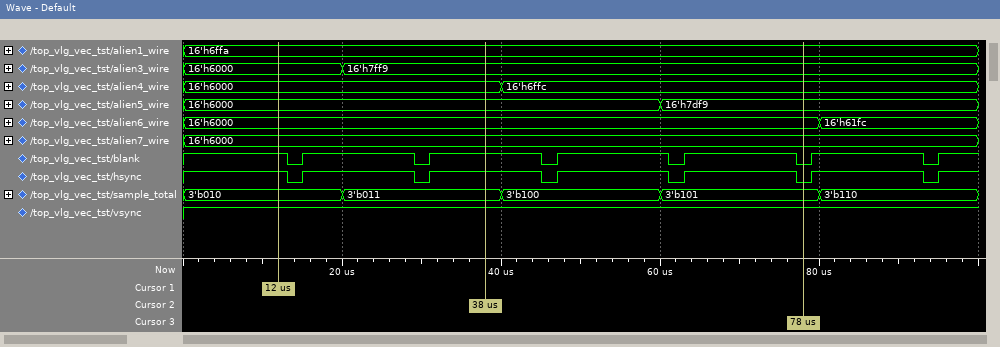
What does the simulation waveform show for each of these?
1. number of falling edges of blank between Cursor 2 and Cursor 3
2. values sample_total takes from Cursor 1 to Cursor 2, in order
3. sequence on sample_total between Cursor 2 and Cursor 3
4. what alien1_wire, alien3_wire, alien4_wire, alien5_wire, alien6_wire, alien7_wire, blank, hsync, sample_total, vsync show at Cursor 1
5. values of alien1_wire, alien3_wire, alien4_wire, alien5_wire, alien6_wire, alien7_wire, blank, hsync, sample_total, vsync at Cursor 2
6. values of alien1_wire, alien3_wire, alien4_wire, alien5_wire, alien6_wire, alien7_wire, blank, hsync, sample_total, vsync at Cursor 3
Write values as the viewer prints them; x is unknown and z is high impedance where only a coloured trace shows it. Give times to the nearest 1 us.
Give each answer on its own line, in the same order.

3
3'b010, 3'b011
3'b011, 3'b100, 3'b101
alien1_wire=16'h6ffa, alien3_wire=16'h6000, alien4_wire=16'h6000, alien5_wire=16'h6000, alien6_wire=16'h6000, alien7_wire=16'h6000, blank=1, hsync=1, sample_total=3'b010, vsync=1
alien1_wire=16'h6ffa, alien3_wire=16'h7ff9, alien4_wire=16'h6000, alien5_wire=16'h6000, alien6_wire=16'h6000, alien7_wire=16'h6000, blank=1, hsync=1, sample_total=3'b011, vsync=1
alien1_wire=16'h6ffa, alien3_wire=16'h7ff9, alien4_wire=16'h6ffc, alien5_wire=16'h7df9, alien6_wire=16'h6000, alien7_wire=16'h6000, blank=0, hsync=0, sample_total=3'b101, vsync=1
